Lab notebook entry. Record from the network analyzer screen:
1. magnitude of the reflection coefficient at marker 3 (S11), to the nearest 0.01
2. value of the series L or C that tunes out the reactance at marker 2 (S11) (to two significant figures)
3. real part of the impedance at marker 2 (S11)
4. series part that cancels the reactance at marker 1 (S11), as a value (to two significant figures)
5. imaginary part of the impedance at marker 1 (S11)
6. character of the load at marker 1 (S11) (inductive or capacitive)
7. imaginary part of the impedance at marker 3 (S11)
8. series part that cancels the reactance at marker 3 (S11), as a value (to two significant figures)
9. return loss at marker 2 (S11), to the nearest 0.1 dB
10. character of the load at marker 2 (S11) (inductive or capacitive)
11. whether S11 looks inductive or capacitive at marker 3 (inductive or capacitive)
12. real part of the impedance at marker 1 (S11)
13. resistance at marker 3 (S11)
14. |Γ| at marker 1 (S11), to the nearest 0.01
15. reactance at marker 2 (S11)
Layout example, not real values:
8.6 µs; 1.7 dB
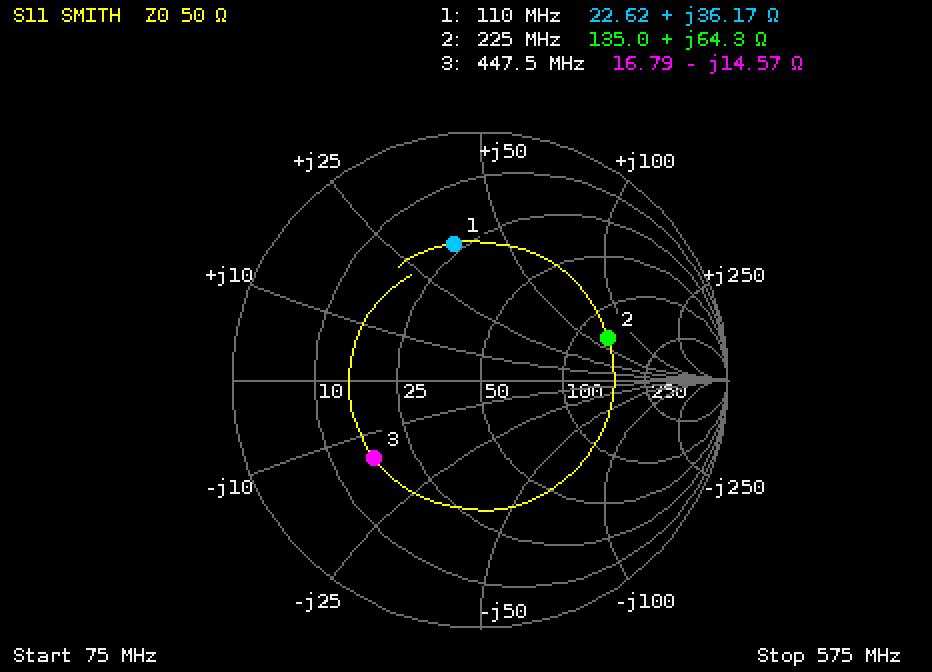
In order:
0.53; 11 pF; 135.0 Ω; 40 pF; +36.17 Ω; inductive; -14.57 Ω; 5.2 nH; 5.3 dB; inductive; capacitive; 22.62 Ω; 16.79 Ω; 0.56; +64.3 Ω
